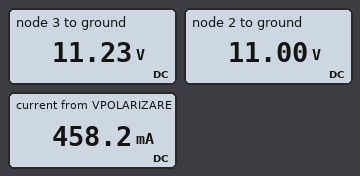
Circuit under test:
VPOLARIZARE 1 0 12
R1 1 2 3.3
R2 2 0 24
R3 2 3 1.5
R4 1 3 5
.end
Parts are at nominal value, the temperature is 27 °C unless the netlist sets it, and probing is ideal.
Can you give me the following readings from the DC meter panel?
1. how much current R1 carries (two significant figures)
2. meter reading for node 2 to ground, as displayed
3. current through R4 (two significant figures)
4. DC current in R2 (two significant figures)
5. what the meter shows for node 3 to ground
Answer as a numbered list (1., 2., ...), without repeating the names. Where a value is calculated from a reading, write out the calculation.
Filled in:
1. (12 V - 11 V) / 3.3 Ω = 300 mA
2. 11.00 V
3. (12 V - 11.23 V) / 5 Ω = 150 mA
4. (11 V) / 24 Ω = 460 mA
5. 11.23 V
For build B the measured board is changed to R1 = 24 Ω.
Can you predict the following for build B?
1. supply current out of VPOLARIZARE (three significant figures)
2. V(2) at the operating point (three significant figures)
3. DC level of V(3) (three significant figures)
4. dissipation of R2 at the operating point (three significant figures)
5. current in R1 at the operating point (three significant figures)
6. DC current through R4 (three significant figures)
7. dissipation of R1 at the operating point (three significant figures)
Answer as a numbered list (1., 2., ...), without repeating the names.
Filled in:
1. 412 mA
2. 9.89 V
3. 10.4 V
4. 4.08 W
5. 87.8 mA
6. 324 mA
7. 185 mW
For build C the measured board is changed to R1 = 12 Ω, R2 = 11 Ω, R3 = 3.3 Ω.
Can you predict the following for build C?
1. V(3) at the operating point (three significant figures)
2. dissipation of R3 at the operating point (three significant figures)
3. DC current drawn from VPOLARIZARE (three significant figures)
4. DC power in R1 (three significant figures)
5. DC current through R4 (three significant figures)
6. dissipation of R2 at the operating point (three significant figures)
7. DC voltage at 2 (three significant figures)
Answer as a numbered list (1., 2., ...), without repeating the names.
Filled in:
1. 9.77 V
2. 656 mW
3. 754 mA
4. 1.14 W
5. 446 mA
6. 6.26 W
7. 8.30 V
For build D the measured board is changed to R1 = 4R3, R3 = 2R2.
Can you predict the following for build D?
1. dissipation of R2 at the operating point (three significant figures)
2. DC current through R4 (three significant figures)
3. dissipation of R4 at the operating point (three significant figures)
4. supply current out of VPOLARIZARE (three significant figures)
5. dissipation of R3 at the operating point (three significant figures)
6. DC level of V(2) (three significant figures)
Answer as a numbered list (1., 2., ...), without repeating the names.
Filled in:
1. 4.85 W
2. 168 mA
3. 141 mW
4. 450 mA
5. 62.2 mW
6. 10.8 V
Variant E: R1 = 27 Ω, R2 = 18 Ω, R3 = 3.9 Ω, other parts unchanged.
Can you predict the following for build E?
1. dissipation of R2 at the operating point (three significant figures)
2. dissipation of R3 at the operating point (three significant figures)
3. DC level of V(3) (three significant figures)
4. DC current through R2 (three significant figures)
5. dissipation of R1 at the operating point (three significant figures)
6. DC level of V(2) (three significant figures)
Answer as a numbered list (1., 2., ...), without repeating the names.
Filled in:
1. 4.25 W
2. 521 mW
3. 10.2 V
4. 486 mA
5. 392 mW
6. 8.75 V
